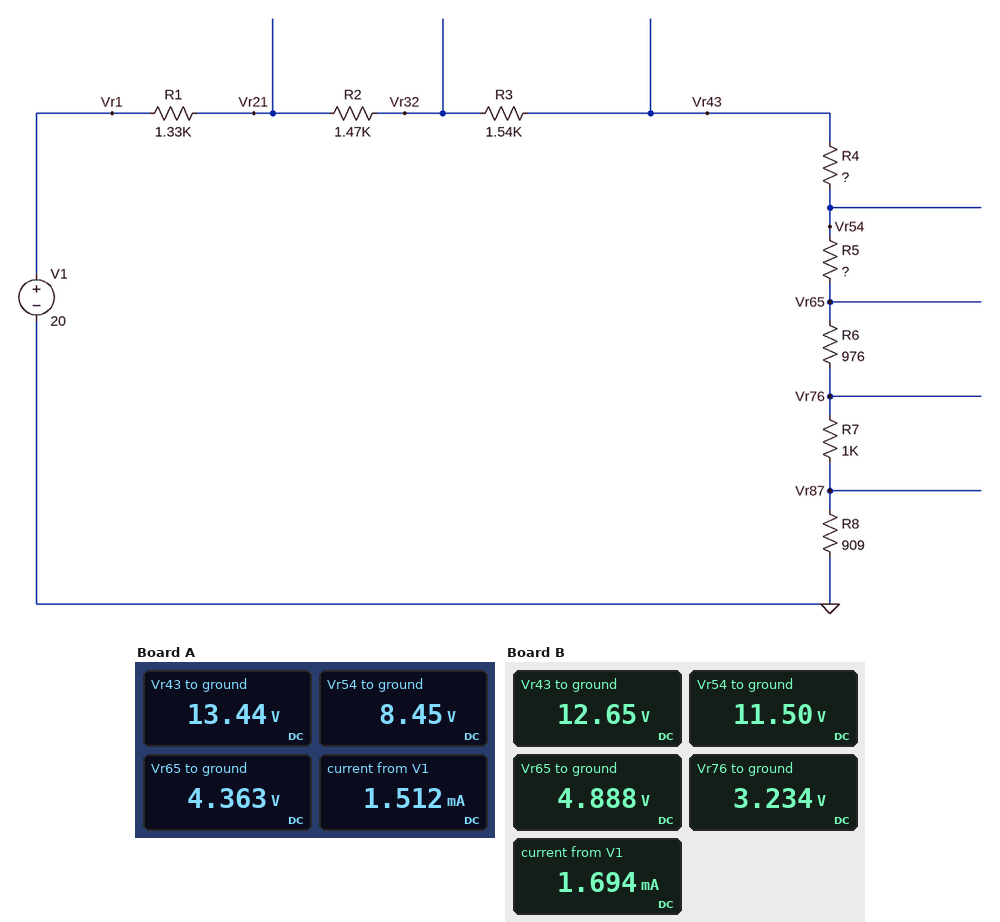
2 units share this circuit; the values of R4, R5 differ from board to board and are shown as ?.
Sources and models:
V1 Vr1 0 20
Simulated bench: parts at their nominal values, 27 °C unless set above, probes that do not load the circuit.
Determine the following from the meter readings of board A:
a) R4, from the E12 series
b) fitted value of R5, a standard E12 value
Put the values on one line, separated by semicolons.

3.3 kΩ; 2.7 kΩ
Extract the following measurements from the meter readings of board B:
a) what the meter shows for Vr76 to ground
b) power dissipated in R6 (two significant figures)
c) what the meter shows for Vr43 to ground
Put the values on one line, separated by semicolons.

3.234 V; 2.8 mW; 12.65 V
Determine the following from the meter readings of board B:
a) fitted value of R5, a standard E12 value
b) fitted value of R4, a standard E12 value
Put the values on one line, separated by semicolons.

3.9 kΩ; 680 Ω
